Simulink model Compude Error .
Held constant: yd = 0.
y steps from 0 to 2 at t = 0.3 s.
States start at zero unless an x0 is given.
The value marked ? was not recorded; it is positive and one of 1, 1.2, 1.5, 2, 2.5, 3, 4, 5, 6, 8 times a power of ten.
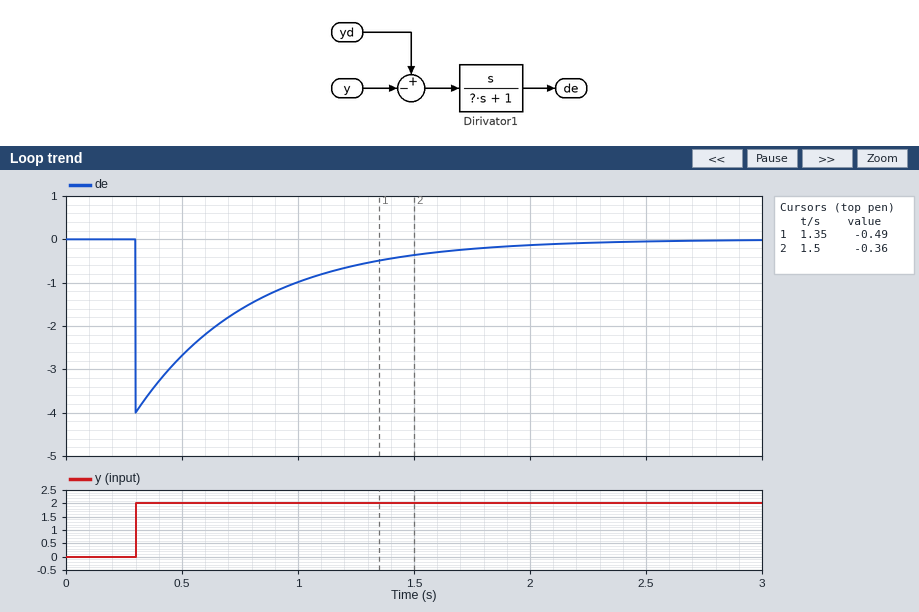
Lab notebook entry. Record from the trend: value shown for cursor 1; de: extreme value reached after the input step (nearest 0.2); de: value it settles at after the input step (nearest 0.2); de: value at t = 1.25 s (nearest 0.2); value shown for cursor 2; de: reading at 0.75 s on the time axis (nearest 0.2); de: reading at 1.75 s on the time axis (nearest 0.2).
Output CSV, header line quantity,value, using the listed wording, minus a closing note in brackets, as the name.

quantity,value
value shown for cursor 1,-0.49
de: extreme value reached after the input step,-4.0
de: value it settles at after the input step,0.0
de: value at t = 1.25 s,-0.6
value shown for cursor 2,-0.36
de: reading at 0.75 s on the time axis,-1.6
de: reading at 1.75 s on the time axis,-0.2
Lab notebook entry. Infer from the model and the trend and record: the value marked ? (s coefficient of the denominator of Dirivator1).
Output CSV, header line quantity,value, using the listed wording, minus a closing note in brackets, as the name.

quantity,value
the value marked ?,0.5
